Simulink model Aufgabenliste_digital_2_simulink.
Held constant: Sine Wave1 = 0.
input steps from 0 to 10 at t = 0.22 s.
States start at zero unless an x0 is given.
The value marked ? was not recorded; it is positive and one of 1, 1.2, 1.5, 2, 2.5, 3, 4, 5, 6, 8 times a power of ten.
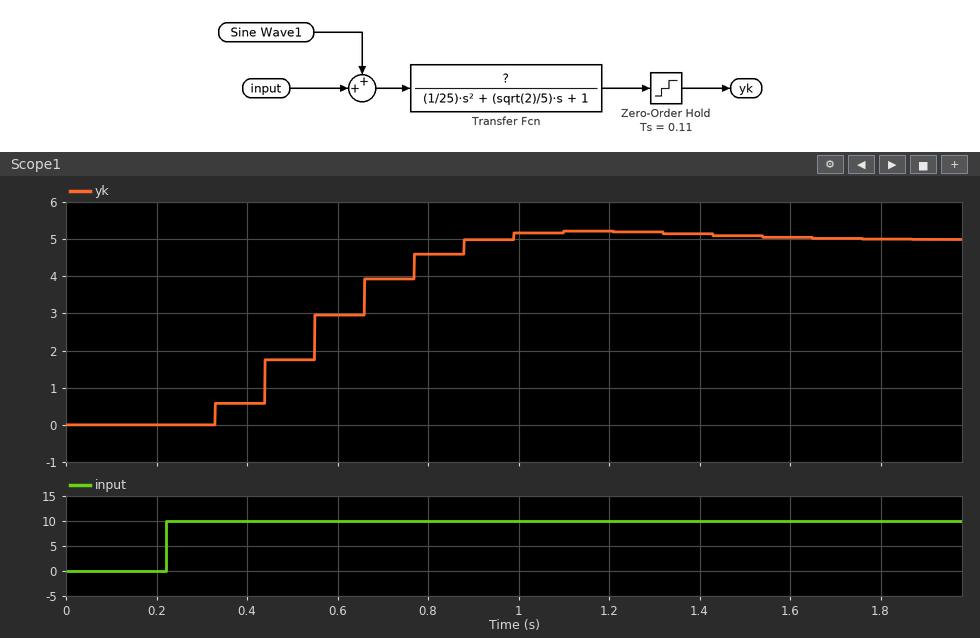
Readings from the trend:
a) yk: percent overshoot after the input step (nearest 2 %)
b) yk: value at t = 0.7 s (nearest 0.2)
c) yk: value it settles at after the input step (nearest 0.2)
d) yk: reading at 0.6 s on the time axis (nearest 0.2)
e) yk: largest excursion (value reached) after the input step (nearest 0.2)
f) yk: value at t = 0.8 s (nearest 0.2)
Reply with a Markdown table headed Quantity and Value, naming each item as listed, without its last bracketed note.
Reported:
| Quantity | Value |
|---|---|
| yk: percent overshoot after the input step | 4 % |
| yk: value at t = 0.7 s | 4.0 |
| yk: value it settles at after the input step | 5.0 |
| yk: reading at 0.6 s on the time axis | 3.0 |
| yk: largest excursion (value reached) after the input step | 5.2 |
| yk: value at t = 0.8 s | 4.6 |
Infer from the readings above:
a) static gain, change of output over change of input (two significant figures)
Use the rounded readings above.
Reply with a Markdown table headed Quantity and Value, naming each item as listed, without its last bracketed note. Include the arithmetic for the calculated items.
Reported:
| Quantity | Value |
|---|---|
| static gain, change of output over change of input | (5 - 0) / (10 - 0) = 0.50 |
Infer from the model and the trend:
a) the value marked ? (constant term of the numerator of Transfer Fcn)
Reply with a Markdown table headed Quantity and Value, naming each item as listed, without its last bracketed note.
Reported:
| Quantity | Value |
|---|---|
| the value marked ? | 0.5 |
